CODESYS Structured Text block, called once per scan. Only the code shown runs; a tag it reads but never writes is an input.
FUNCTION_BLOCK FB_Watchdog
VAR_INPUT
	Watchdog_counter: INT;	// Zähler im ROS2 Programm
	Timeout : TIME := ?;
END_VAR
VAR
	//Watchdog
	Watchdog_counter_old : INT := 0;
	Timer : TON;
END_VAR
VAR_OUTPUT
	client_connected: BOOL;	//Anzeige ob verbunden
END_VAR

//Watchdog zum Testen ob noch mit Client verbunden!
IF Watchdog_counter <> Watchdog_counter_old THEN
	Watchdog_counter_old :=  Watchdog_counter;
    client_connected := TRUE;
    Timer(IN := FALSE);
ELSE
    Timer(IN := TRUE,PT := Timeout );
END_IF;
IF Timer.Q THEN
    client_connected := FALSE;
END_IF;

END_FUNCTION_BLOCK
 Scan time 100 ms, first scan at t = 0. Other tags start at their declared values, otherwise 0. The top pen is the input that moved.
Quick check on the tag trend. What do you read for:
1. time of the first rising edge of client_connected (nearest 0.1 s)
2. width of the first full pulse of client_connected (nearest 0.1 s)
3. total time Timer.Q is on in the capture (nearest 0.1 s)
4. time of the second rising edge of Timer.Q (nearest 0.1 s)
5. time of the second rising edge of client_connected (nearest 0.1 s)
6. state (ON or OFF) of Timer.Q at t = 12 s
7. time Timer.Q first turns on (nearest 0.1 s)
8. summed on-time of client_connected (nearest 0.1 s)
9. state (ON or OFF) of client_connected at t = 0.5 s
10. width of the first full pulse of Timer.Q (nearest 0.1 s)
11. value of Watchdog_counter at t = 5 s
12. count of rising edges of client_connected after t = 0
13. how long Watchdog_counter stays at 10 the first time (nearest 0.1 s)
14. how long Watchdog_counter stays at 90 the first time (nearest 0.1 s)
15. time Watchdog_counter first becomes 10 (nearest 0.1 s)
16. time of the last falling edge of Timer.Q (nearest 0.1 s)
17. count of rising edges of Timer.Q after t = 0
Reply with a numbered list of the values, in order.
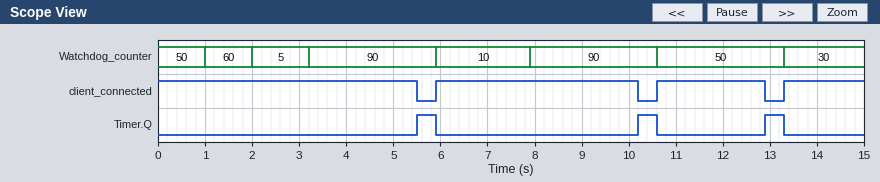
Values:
1. 5.9 s
2. 4.3 s
3. 1.2 s
4. 10.2 s
5. 10.6 s
6. OFF
7. 5.5 s
8. 13.8 s
9. ON
10. 0.4 s
11. 90
12. 3
13. 2.0 s
14. 2.7 s
15. 5.9 s
16. 13.3 s
17. 3
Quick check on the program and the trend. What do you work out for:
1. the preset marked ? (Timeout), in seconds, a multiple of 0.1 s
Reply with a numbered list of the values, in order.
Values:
1. 2.2 s
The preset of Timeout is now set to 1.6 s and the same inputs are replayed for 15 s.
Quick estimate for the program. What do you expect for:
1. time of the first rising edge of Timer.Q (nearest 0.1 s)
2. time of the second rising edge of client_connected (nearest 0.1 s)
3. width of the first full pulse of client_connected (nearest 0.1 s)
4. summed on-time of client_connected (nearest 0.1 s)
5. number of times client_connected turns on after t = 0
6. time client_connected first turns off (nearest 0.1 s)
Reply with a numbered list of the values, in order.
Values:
1. 4.9 s
2. 7.9 s
3. 1.7 s
4. 11.7 s
5. 4
6. 4.9 s
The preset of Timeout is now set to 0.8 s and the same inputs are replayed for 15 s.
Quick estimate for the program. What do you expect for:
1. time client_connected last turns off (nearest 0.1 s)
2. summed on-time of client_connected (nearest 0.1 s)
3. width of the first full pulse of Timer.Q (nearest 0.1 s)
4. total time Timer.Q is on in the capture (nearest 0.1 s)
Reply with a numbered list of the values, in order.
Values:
1. 14.2 s
2. 7.2 s
3. 0.1 s
4. 7.8 s
